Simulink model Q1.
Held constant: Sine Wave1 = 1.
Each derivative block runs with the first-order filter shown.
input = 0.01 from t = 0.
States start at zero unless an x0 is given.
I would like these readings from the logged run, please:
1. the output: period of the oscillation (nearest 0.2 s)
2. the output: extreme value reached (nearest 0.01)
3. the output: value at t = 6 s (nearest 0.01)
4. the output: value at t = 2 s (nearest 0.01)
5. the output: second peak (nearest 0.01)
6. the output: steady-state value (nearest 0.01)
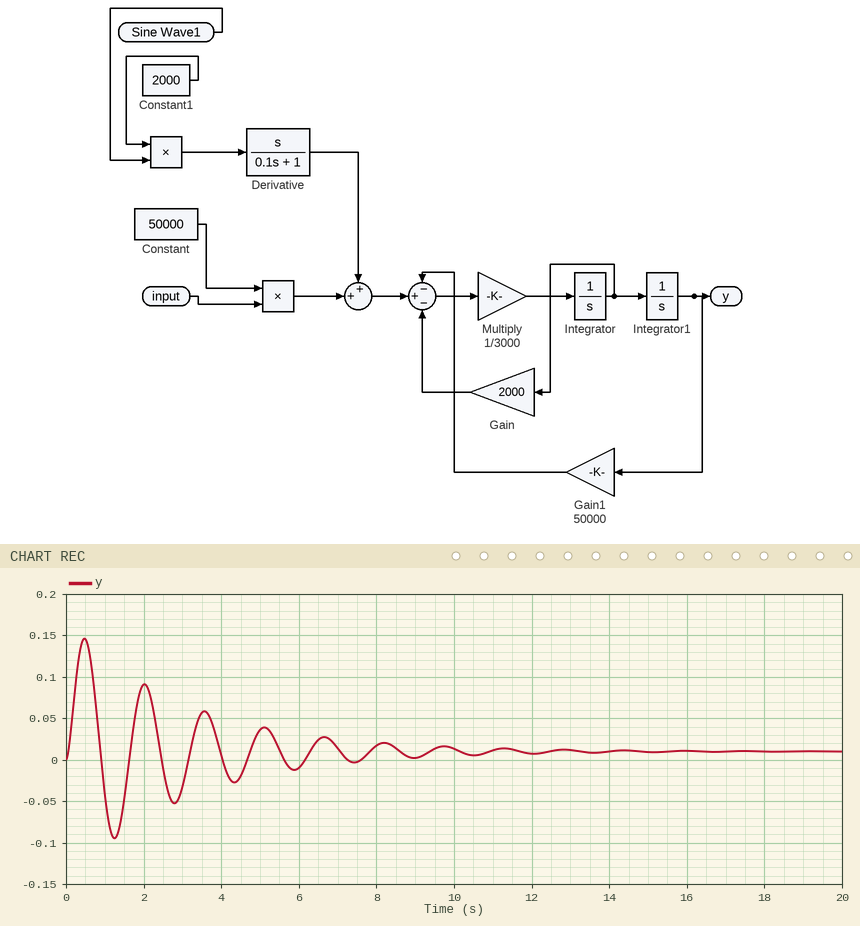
1.6 s
0.15
-0.01
0.09
0.09
0.01
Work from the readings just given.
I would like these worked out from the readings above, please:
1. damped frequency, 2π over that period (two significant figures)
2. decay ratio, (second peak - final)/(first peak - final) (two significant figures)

3.9 rad/s
0.57
